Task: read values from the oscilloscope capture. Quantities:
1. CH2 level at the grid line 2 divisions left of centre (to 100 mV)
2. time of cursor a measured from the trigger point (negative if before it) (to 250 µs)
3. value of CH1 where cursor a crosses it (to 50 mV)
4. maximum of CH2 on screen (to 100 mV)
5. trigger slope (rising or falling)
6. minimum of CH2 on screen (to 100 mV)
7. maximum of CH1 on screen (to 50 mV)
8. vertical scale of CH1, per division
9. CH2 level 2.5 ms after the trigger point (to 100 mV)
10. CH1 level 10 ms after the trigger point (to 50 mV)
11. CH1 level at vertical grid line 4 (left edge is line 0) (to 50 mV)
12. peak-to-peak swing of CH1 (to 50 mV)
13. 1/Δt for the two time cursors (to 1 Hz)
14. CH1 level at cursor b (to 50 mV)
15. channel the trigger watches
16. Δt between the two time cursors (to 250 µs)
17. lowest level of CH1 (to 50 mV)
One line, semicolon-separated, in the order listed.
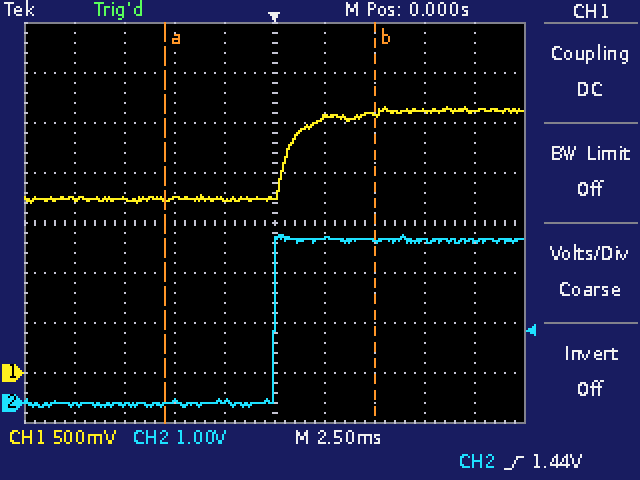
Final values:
0.0 V; -5.50 ms; 1.75 V; 3.4 V; rising; -100 mV; 2.65 V; 500 mV; 3.3 V; 2.60 V; 1.75 V; 950 mV; 95 Hz; 2.60 V; CH2; 10.50 ms; 1.70 V
